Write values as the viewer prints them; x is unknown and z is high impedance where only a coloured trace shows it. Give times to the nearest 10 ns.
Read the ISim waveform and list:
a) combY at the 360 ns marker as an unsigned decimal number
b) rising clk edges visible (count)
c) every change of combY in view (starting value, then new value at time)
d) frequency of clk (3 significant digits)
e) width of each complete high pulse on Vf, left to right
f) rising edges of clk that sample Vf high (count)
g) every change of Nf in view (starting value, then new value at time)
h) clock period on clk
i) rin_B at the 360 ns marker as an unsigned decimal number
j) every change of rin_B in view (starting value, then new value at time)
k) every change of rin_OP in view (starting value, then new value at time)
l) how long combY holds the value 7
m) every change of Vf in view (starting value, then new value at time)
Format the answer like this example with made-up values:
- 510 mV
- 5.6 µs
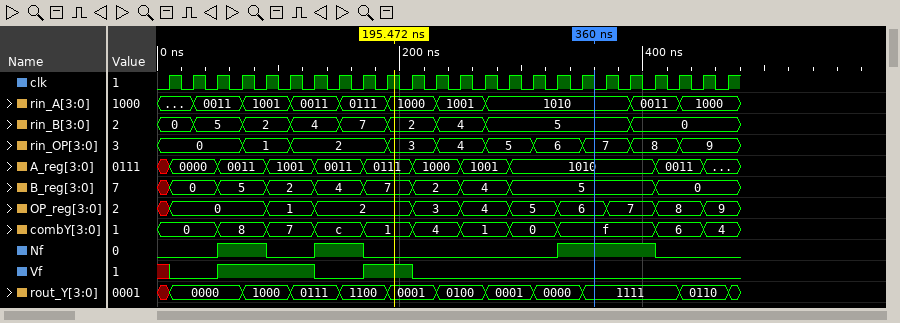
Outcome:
- 15
- 24
- 0, 8 at 50 ns, 7 at 90 ns, c at 130 ns, 1 at 170 ns, 4 at 210 ns, 1 at 250 ns, 0 at 290 ns, f at 330 ns, 6 at 410 ns, 4 at 450 ns
- 50.0 MHz
- 80 ns, 40 ns
- 6
- 0, 1 at 50 ns, 0 at 90 ns, 1 at 130 ns, 0 at 170 ns, 1 at 330 ns, 0 at 410 ns
- 20 ns
- 5
- 0, 5 at 30 ns, 2 at 70 ns, 4 at 110 ns, 7 at 150 ns, 2 at 190 ns, 4 at 230 ns, 5 at 270 ns, 0 at 390 ns
- 0, 1 at 70 ns, 2 at 110 ns, 3 at 190 ns, 4 at 230 ns, 5 at 270 ns, 6 at 310 ns, 7 at 350 ns, 8 at 390 ns, 9 at 430 ns
- 40 ns
- x, 0 at 10 ns, 1 at 50 ns, 0 at 130 ns, 1 at 170 ns, 0 at 210 ns
